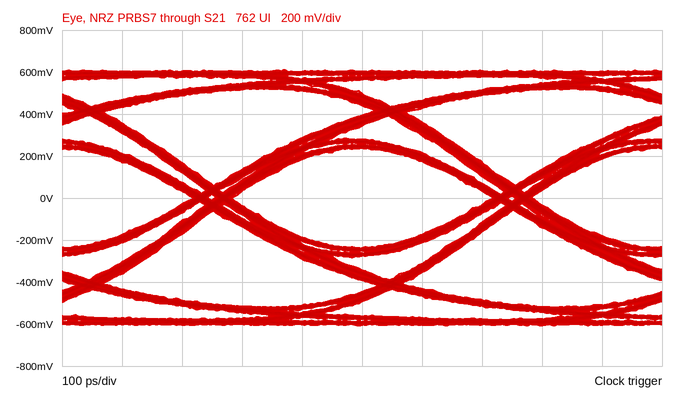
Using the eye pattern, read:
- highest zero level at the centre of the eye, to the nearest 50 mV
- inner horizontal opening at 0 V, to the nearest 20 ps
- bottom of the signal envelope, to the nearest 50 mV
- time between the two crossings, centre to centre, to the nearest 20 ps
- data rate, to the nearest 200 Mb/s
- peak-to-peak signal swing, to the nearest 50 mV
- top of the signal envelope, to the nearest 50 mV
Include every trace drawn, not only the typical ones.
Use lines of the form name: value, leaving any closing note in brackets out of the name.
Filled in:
highest zero level at the centre of the eye, to the nearest 50 mV: -250 mV
inner horizontal opening at 0 V, to the nearest 20 ps: 440 ps
bottom of the signal envelope, to the nearest 50 mV: -600 mV
time between the two crossings, centre to centre, to the nearest 20 ps: 500 ps
data rate, to the nearest 200 Mb/s: 2.0 Gb/s
peak-to-peak signal swing, to the nearest 50 mV: 1.20 V
top of the signal envelope, to the nearest 50 mV: 600 mV
